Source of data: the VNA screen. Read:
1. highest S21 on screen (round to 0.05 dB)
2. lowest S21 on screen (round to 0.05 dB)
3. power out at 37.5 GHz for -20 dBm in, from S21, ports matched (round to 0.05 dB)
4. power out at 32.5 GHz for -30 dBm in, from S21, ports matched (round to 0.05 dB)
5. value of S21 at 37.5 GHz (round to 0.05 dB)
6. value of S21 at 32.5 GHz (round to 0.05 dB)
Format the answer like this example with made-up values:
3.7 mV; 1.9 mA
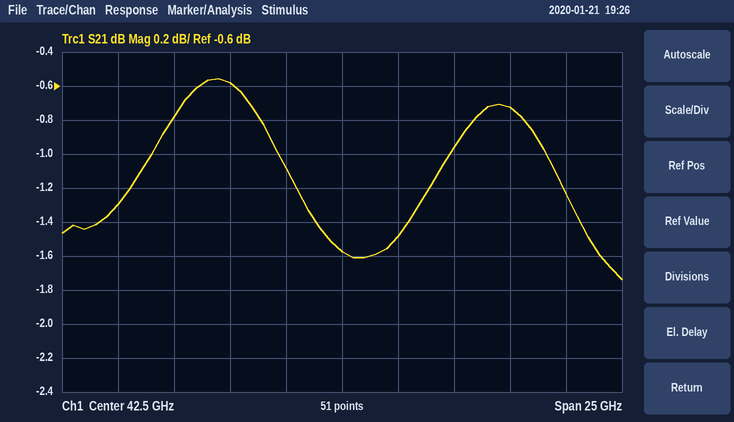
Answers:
-0.55 dB; -1.75 dB; -20.60 dBm; -31.30 dBm; -0.60 dB; -1.30 dB
